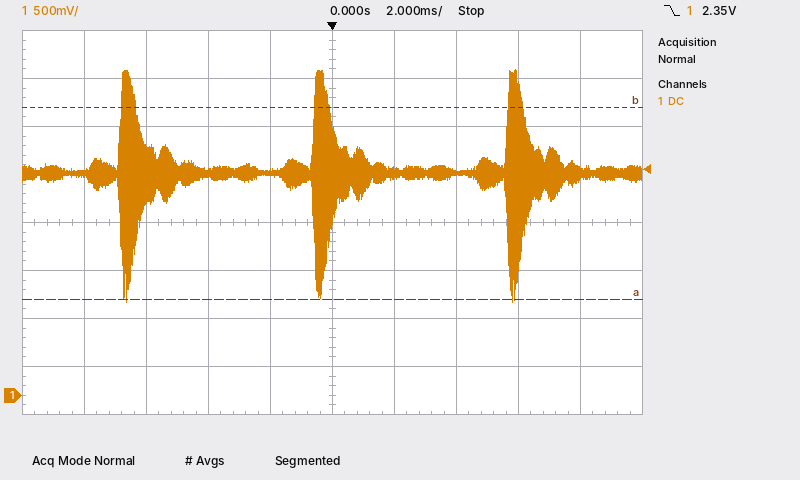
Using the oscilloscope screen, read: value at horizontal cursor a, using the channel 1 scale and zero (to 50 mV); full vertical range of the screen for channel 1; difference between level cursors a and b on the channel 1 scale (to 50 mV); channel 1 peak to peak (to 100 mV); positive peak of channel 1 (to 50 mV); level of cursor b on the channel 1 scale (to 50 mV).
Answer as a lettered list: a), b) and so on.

a) 1.00 V
b) 4 V
c) 2.00 V
d) 2.40 V
e) 3.40 V
f) 3.00 V
